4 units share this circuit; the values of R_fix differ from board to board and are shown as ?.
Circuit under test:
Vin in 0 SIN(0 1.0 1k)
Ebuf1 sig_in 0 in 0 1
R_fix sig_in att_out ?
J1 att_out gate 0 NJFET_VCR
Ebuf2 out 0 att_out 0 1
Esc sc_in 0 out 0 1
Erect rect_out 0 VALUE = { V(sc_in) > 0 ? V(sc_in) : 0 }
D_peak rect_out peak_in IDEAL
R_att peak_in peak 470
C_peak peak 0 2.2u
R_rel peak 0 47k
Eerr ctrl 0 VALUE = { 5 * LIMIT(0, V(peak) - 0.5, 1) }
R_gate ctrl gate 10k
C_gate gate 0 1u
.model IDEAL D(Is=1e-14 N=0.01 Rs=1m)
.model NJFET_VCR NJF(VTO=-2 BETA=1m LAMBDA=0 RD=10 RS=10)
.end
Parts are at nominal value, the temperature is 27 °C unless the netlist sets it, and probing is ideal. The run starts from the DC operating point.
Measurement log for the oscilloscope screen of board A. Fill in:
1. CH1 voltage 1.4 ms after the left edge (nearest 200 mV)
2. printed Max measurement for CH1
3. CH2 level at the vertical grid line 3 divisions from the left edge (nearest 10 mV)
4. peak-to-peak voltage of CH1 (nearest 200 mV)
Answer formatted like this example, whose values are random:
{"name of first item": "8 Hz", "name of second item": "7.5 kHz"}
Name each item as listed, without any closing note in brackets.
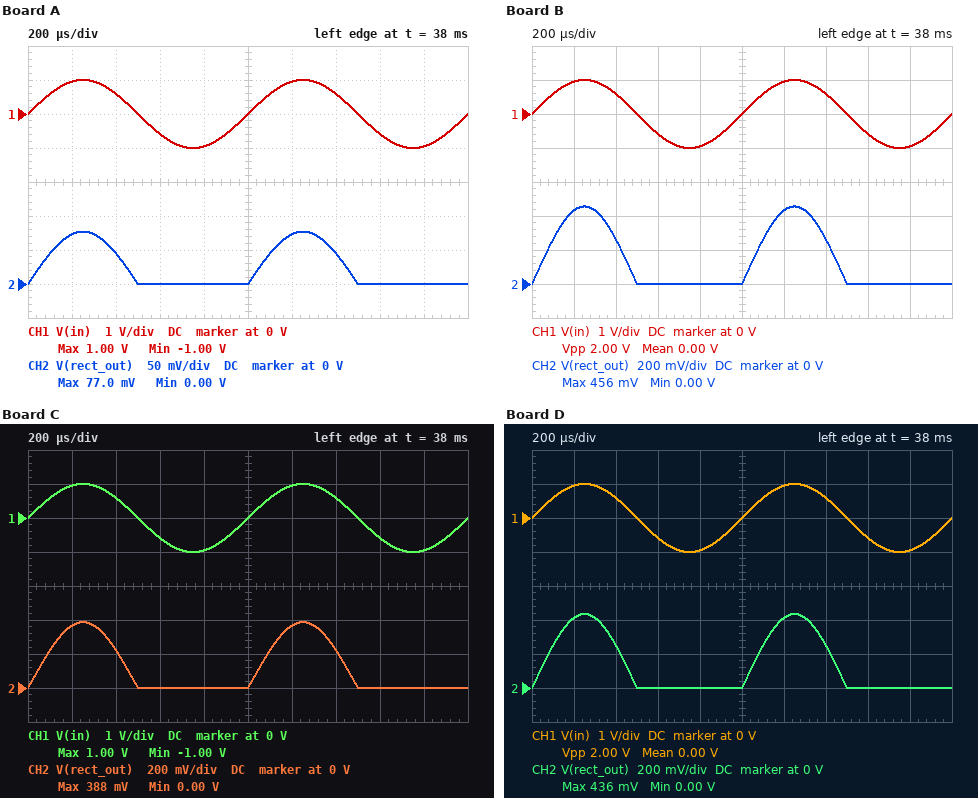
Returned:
{"CH1 voltage 1.4 ms after the left edge": "600 mV", "printed Max measurement for CH1": "1.00 V", "CH2 level at the vertical grid line 3 divisions from the left edge": "0 V", "peak-to-peak voltage of CH1": "2.0 V"}
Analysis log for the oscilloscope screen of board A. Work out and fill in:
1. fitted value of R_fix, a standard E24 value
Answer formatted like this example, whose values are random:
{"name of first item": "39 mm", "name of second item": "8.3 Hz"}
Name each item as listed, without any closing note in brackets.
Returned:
{"fitted value of R_fix, a standard E24 value": "3.3 kΩ"}
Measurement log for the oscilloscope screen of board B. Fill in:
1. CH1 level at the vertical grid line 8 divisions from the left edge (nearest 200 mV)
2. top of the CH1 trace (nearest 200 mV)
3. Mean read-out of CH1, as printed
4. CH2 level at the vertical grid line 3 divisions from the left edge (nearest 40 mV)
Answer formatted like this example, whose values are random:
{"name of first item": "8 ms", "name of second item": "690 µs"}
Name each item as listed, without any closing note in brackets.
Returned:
{"CH1 level at the vertical grid line 8 divisions from the left edge": "-600 mV", "top of the CH1 trace": "1.0 V", "Mean read-out of CH1, as printed": "0.00 V", "CH2 level at the vertical grid line 3 divisions from the left edge": "0 V"}
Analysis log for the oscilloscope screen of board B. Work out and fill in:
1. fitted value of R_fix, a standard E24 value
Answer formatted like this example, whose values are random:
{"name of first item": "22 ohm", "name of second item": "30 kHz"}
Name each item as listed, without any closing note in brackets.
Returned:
{"fitted value of R_fix, a standard E24 value": "360 Ω"}
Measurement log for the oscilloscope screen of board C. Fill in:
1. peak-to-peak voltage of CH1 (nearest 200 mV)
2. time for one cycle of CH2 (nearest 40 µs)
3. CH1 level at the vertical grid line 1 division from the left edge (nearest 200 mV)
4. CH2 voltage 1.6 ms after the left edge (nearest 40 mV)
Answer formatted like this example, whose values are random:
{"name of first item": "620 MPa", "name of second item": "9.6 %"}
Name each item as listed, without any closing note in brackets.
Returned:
{"peak-to-peak voltage of CH1": "2.0 V", "time for one cycle of CH2": "1.00 ms", "CH1 level at the vertical grid line 1 division from the left edge": "1.0 V", "CH2 voltage 1.6 ms after the left edge": "0 V"}
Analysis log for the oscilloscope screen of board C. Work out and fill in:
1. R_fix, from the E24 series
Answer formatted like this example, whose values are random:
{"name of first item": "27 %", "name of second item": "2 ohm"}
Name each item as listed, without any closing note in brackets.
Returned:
{"R_fix, from the E24 series": "470 Ω"}
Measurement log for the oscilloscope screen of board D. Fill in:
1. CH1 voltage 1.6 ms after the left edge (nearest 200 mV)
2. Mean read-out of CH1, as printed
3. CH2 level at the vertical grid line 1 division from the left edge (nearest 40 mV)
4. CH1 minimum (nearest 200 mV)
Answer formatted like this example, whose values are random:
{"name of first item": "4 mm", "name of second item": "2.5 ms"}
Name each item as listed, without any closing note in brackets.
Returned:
{"CH1 voltage 1.6 ms after the left edge": "-600 mV", "Mean read-out of CH1, as printed": "0.00 V", "CH2 level at the vertical grid line 1 division from the left edge": "400 mV", "CH1 minimum": "-1.0 V"}
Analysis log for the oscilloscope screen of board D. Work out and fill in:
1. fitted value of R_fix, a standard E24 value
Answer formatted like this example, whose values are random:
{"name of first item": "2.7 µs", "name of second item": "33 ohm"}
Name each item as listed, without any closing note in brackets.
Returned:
{"fitted value of R_fix, a standard E24 value": "390 Ω"}
